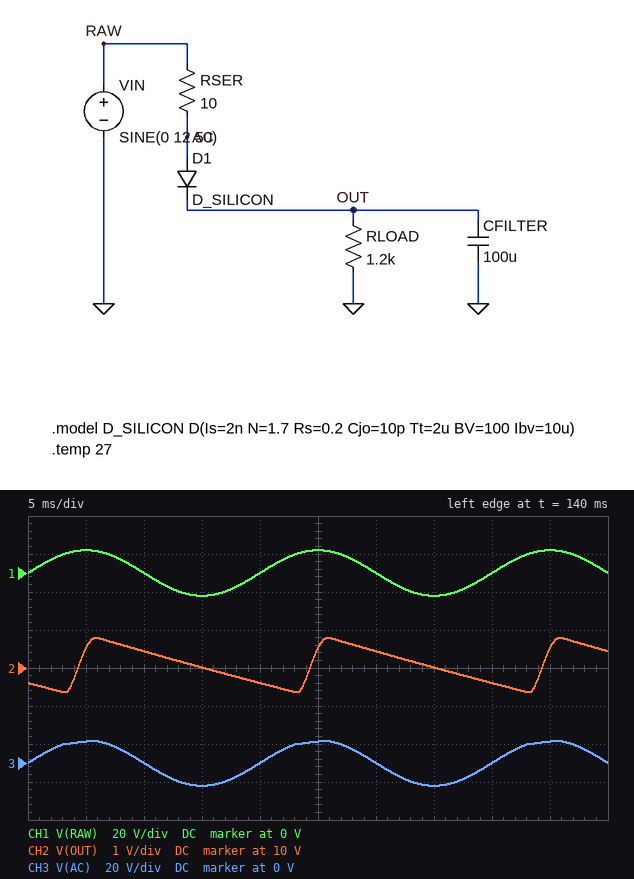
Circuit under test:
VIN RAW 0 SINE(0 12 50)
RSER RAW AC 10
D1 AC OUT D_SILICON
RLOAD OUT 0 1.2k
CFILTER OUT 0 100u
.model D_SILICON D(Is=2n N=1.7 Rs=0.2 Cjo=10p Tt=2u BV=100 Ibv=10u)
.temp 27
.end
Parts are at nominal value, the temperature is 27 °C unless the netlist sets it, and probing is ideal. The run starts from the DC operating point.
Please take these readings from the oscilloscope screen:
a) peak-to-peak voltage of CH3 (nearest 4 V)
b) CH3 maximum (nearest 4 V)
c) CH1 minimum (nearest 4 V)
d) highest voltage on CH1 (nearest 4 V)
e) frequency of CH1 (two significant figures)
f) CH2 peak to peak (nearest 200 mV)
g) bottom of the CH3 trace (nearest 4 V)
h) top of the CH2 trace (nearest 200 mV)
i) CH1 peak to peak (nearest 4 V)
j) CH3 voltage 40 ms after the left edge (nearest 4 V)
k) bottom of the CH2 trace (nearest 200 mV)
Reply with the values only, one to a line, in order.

24 V
12 V
-12 V
12 V
50 Hz
1.4 V
-12 V
10.8 V
24 V
0 V
9.4 V
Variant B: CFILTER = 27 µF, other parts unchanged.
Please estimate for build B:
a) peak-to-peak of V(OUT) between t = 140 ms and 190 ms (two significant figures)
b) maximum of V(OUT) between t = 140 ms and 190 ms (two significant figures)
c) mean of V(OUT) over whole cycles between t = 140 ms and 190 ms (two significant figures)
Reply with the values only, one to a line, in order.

4.5 V
11 V
8.9 V
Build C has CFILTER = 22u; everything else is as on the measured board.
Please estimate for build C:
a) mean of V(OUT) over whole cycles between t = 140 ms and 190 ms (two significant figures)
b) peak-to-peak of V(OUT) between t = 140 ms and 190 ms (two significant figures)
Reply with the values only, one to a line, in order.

8.5 V
5.2 V
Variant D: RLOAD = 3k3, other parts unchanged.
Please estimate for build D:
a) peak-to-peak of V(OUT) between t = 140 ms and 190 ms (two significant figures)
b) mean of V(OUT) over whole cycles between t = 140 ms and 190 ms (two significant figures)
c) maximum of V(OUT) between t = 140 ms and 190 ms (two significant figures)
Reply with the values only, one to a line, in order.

580 mV
11 V
11 V
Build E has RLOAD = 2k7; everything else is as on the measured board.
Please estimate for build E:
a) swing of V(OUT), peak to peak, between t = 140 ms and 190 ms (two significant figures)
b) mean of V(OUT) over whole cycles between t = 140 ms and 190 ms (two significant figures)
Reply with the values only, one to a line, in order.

700 mV
11 V
